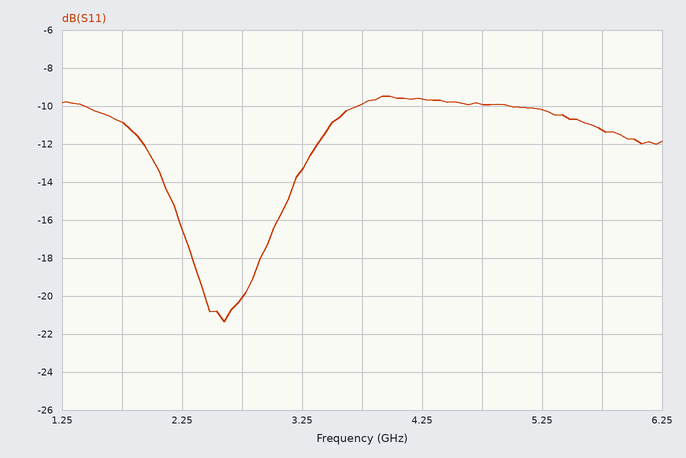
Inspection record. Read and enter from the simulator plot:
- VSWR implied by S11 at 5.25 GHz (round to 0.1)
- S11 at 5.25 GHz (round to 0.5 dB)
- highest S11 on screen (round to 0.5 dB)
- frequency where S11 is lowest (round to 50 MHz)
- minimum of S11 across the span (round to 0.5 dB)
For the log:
1.9
-10.0 dB
-9.5 dB
2.60 GHz
-21.5 dB
